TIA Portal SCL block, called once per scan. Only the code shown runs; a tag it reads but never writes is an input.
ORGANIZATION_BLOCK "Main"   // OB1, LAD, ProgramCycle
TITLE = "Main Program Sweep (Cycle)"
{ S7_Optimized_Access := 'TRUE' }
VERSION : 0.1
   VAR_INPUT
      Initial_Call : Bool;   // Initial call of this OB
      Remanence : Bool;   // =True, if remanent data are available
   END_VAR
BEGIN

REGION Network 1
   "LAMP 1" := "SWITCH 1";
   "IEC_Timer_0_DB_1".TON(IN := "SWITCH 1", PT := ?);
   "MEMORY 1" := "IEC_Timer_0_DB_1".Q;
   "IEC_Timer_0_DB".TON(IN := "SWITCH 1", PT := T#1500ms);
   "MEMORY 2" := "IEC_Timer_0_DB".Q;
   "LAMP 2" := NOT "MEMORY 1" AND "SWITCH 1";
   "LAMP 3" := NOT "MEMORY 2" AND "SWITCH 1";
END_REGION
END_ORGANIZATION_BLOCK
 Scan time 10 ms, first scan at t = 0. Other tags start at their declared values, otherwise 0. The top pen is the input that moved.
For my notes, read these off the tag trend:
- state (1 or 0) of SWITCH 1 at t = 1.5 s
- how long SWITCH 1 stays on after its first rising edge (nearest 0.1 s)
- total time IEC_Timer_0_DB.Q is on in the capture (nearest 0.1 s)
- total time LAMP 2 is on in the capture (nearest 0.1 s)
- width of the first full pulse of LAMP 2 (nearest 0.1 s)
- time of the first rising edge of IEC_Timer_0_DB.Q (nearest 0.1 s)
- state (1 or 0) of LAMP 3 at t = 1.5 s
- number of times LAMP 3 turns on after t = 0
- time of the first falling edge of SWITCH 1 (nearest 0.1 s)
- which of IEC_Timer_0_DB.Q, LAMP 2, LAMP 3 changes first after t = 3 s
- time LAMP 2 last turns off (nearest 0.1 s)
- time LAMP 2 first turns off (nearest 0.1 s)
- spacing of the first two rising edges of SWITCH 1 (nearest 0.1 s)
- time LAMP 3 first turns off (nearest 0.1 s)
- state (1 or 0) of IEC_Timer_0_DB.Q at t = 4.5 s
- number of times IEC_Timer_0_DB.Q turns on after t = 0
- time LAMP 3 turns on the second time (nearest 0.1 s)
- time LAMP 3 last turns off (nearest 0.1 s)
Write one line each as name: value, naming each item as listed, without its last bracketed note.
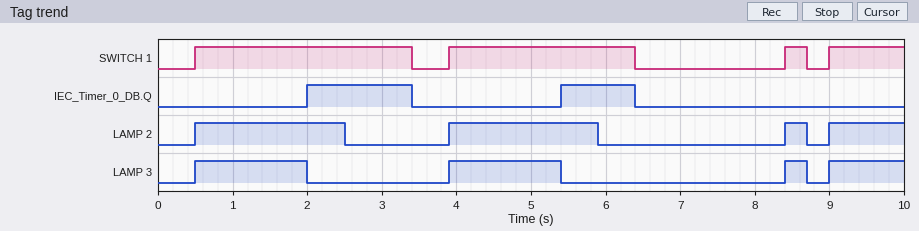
state (1 or 0) of SWITCH 1 at t = 1.5 s: 1
how long SWITCH 1 stays on after its first rising edge: 2.9 s
total time IEC_Timer_0_DB.Q is on in the capture: 2.4 s
total time LAMP 2 is on in the capture: 5.3 s
width of the first full pulse of LAMP 2: 2.0 s
time of the first rising edge of IEC_Timer_0_DB.Q: 2.0 s
state (1 or 0) of LAMP 3 at t = 1.5 s: 1
number of times LAMP 3 turns on after t = 0: 4
time of the first falling edge of SWITCH 1: 3.4 s
which of IEC_Timer_0_DB.Q, LAMP 2, LAMP 3 changes first after t = 3 s: IEC_Timer_0_DB.Q
time LAMP 2 last turns off: 8.7 s
time LAMP 2 first turns off: 2.5 s
spacing of the first two rising edges of SWITCH 1: 3.4 s
time LAMP 3 first turns off: 2.0 s
state (1 or 0) of IEC_Timer_0_DB.Q at t = 4.5 s: 0
number of times IEC_Timer_0_DB.Q turns on after t = 0: 2
time LAMP 3 turns on the second time: 3.9 s
time LAMP 3 last turns off: 8.7 s
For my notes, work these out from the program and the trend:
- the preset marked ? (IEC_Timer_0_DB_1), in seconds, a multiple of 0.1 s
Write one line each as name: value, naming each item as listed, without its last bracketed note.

the preset marked ? (IEC_Timer_0_DB_1), in seconds, a multiple of 0.1 s: 2.0 s
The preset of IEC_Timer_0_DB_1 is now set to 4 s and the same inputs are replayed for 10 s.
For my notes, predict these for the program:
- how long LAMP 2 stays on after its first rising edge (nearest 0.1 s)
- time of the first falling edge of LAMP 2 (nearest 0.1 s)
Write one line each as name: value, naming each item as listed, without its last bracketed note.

how long LAMP 2 stays on after its first rising edge: 2.9 s
time of the first falling edge of LAMP 2: 3.4 s
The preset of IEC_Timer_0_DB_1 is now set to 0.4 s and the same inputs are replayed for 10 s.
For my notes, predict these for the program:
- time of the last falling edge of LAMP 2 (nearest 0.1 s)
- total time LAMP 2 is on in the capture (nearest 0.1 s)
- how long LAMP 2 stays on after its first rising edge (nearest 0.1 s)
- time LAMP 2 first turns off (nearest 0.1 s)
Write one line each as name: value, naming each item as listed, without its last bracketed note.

time of the last falling edge of LAMP 2: 9.4 s
total time LAMP 2 is on in the capture: 1.5 s
how long LAMP 2 stays on after its first rising edge: 0.4 s
time LAMP 2 first turns off: 0.9 s
